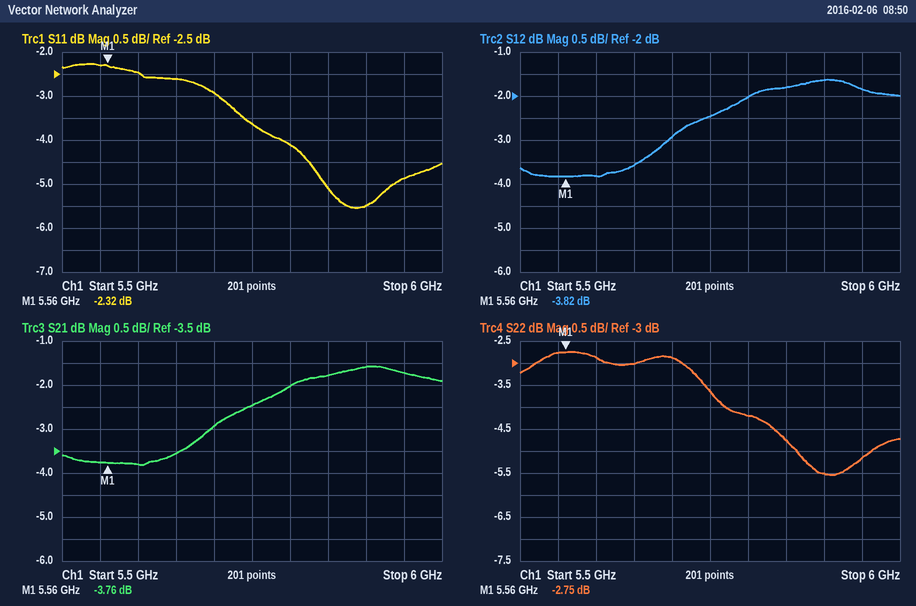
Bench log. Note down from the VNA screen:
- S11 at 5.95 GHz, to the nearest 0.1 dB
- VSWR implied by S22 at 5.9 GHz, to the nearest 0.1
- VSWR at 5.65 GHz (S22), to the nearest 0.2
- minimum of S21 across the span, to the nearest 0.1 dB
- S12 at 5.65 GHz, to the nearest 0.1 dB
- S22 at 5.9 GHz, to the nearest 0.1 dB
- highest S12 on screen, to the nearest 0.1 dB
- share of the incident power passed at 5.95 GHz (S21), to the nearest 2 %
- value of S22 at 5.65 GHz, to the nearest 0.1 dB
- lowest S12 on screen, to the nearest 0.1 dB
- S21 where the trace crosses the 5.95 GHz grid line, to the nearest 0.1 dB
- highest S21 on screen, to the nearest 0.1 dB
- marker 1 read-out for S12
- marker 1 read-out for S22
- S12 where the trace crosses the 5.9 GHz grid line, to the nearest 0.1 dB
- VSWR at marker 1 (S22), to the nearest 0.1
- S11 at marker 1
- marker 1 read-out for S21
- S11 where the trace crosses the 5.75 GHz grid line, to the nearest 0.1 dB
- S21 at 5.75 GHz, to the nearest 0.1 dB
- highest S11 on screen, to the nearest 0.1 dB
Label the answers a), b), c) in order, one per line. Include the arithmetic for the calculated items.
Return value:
a) -4.9 dB
b) |Γ| = 10^(-5.5/20) = 0.5309; VSWR = (1 + 0.5309)/(1 − 0.5309) ≈ 3.3
c) |Γ| = 10^(-3/20) = 0.7079; VSWR = (1 + 0.7079)/(1 − 0.7079) ≈ 5.8
d) -3.8 dB
e) -3.6 dB
f) -5.5 dB
g) -1.6 dB
h) 10^(-1.7/10) ≈ 68 %
i) -3.0 dB
j) -3.8 dB
k) -1.7 dB
l) -1.6 dB
m) -3.82 dB
n) -2.75 dB
o) -1.6 dB
p) (1 + 0.7286)/(1 − 0.7286) ≈ 6.4
q) -2.32 dB
r) -3.76 dB
s) -3.6 dB
t) -2.5 dB
u) -2.3 dB
